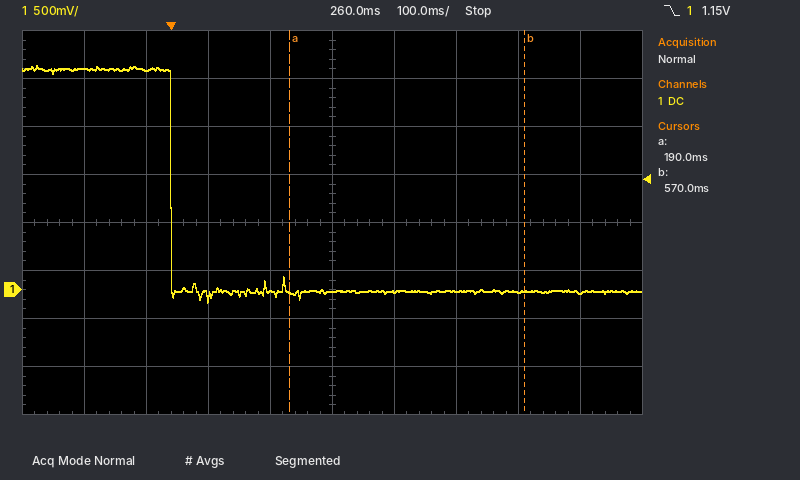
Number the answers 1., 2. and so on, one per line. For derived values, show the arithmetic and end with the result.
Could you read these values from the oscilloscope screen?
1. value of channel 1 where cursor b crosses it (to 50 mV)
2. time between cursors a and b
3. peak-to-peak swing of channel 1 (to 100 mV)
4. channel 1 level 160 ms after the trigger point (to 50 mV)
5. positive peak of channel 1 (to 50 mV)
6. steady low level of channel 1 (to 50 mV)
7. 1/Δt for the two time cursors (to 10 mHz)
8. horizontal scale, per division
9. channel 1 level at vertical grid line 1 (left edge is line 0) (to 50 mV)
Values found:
1. 0 mV
2. 570 ms − (190 ms) = 380 ms
3. 2.50 V
4. 0 mV
5. 2.35 V
6. 0 mV
7. 1 / 380 ms ≈ 2.63 Hz
8. 100 ms
9. 2.30 V
